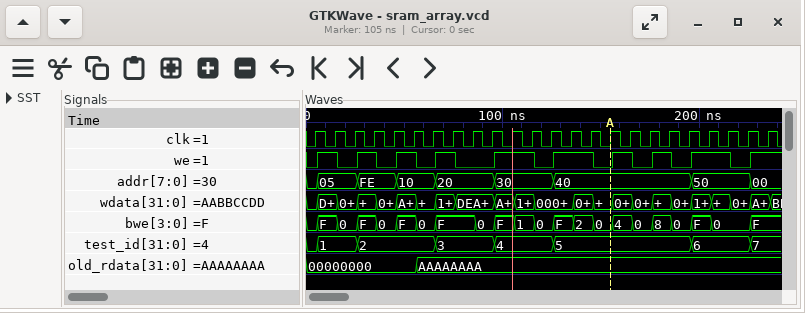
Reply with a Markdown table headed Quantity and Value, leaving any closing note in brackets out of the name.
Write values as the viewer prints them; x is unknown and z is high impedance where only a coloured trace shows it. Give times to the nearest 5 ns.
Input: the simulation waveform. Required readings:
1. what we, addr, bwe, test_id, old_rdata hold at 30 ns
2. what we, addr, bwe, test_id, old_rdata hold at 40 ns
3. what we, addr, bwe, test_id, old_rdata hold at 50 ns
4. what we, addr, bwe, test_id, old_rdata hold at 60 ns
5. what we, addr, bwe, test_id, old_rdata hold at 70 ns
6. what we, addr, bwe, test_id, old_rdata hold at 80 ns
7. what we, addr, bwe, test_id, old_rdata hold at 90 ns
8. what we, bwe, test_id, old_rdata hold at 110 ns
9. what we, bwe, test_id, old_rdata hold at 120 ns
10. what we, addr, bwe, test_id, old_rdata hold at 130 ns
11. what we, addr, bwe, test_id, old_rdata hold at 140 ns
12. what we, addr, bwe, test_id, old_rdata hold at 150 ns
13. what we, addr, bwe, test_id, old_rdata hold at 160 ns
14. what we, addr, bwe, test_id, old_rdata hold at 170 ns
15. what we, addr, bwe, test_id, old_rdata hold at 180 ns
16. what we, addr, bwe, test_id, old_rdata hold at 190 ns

| Quantity | Value |
|---|---|
| what we, addr, bwe, test_id, old_rdata hold at 30 ns | we=1, addr=FE, bwe=F, test_id=2, old_rdata=00000000 |
| what we, addr, bwe, test_id, old_rdata hold at 40 ns | we=0, addr=FE, bwe=0, test_id=2, old_rdata=00000000 |
| what we, addr, bwe, test_id, old_rdata hold at 50 ns | we=1, addr=10, bwe=F, test_id=2, old_rdata=00000000 |
| what we, addr, bwe, test_id, old_rdata hold at 60 ns | we=0, addr=10, bwe=0, test_id=2, old_rdata=AAAAAAAA |
| what we, addr, bwe, test_id, old_rdata hold at 70 ns | we=1, addr=20, bwe=F, test_id=3, old_rdata=AAAAAAAA |
| what we, addr, bwe, test_id, old_rdata hold at 80 ns | we=0, addr=20, bwe=F, test_id=3, old_rdata=AAAAAAAA |
| what we, addr, bwe, test_id, old_rdata hold at 90 ns | we=0, addr=20, bwe=0, test_id=3, old_rdata=AAAAAAAA |
| what we, bwe, test_id, old_rdata hold at 110 ns | we=1, bwe=1, test_id=4, old_rdata=AAAAAAAA |
| what we, bwe, test_id, old_rdata hold at 120 ns | we=0, bwe=0, test_id=4, old_rdata=AAAAAAAA |
| what we, addr, bwe, test_id, old_rdata hold at 130 ns | we=1, addr=40, bwe=F, test_id=5, old_rdata=AAAAAAAA |
| what we, addr, bwe, test_id, old_rdata hold at 140 ns | we=1, addr=40, bwe=2, test_id=5, old_rdata=AAAAAAAA |
| what we, addr, bwe, test_id, old_rdata hold at 150 ns | we=0, addr=40, bwe=0, test_id=5, old_rdata=AAAAAAAA |
| what we, addr, bwe, test_id, old_rdata hold at 160 ns | we=1, addr=40, bwe=4, test_id=5, old_rdata=AAAAAAAA |
| what we, addr, bwe, test_id, old_rdata hold at 170 ns | we=0, addr=40, bwe=0, test_id=5, old_rdata=AAAAAAAA |
| what we, addr, bwe, test_id, old_rdata hold at 180 ns | we=1, addr=40, bwe=8, test_id=5, old_rdata=AAAAAAAA |
| what we, addr, bwe, test_id, old_rdata hold at 190 ns | we=0, addr=40, bwe=0, test_id=5, old_rdata=AAAAAAAA |
